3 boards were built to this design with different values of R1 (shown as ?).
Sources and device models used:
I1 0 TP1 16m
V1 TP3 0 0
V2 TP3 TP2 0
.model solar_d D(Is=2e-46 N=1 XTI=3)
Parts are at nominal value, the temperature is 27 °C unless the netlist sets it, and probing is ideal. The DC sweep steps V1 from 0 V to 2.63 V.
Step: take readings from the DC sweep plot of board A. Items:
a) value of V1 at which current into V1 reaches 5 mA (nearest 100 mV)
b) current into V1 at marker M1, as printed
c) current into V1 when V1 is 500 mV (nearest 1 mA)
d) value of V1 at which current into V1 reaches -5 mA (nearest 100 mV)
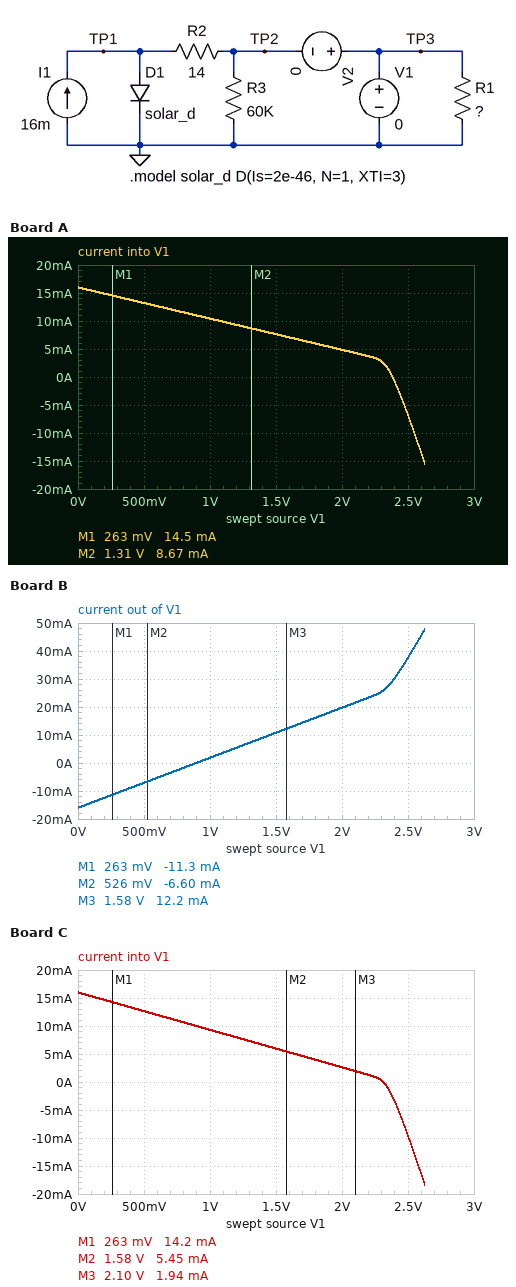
2.0 V
14.5 mA
13 mA
2.5 V
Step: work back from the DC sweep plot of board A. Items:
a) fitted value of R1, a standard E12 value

180 Ω
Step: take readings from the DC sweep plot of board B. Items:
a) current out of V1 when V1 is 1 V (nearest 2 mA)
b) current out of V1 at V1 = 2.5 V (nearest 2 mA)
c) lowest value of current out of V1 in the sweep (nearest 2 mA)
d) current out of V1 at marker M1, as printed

2 mA
38 mA
-16 mA
-11.3 mA
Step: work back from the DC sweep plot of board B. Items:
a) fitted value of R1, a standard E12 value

56 Ω
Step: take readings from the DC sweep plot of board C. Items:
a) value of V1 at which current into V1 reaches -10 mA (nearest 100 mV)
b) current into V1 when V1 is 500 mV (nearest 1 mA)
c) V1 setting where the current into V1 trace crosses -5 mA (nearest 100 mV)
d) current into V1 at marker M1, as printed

2.5 V
13 mA
2.4 V
14.2 mA
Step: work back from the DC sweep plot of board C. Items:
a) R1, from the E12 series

150 Ω
